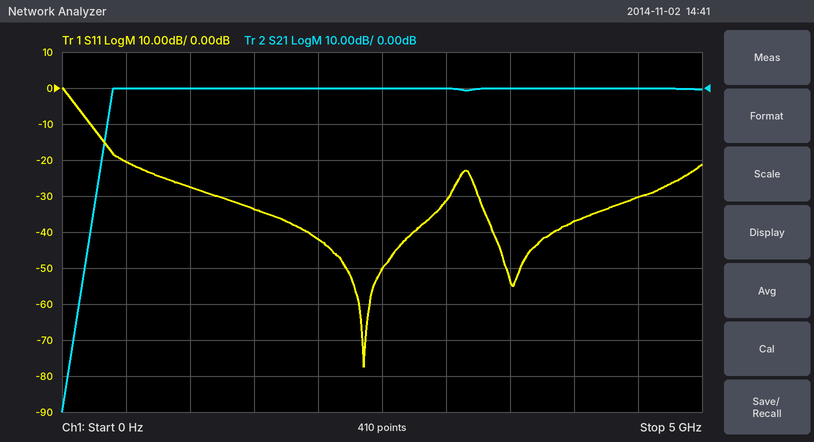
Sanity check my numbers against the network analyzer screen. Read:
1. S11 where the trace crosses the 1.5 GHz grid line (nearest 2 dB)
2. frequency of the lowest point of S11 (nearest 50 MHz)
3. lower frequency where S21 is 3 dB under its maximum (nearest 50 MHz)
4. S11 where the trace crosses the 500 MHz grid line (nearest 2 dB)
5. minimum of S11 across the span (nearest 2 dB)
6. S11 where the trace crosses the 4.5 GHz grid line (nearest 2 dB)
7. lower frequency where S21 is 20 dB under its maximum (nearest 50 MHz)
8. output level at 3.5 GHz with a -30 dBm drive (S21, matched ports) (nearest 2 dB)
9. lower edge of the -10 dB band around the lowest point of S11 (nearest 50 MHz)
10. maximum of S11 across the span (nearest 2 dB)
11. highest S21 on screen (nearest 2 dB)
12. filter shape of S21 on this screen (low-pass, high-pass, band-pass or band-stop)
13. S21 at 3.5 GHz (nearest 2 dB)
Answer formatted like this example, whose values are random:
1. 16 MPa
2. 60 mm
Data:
1. -34 dB
2. 2.35 GHz
3. 400 MHz
4. -20 dB
5. -78 dB
6. -30 dB
7. 300 MHz
8. -30 dBm
9. 200 MHz
10. 0 dB
11. 0 dB
12. high-pass
13. 0 dB
